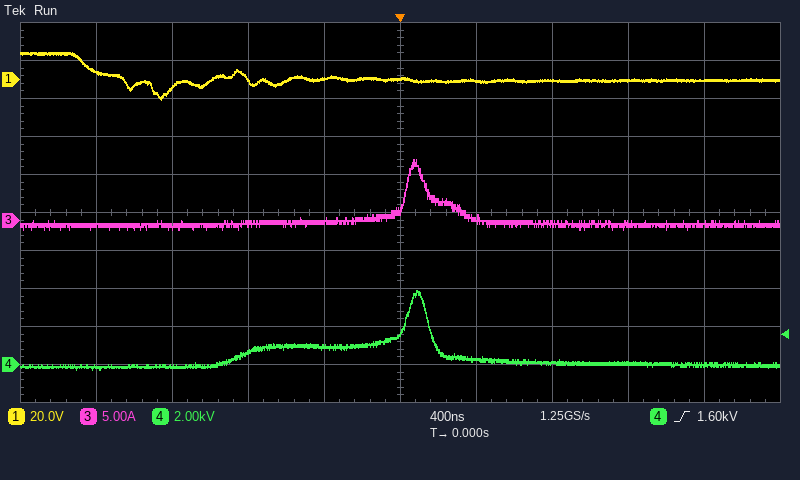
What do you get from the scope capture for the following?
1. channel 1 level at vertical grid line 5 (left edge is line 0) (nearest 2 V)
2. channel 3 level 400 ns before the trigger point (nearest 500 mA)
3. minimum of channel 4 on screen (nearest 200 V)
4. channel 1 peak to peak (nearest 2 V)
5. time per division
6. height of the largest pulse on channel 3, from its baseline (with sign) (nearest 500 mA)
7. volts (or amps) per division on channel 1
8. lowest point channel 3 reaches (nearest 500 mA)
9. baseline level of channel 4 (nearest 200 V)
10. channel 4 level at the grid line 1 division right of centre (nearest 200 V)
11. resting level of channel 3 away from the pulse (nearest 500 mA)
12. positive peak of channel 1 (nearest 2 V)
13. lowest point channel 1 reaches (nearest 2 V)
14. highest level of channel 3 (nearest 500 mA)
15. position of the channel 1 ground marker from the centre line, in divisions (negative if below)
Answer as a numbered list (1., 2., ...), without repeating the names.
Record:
1. 0 V
2. 0.0 A
3. -200 V
4. 24 V
5. 400 ns
6. +8.5 A
7. 20 V
8. -1.0 A
9. 0.0 kV
10. 200 V
11. -500 mA
12. 14 V
13. -10 V
14. 8.0 A
15. +3.5 div
